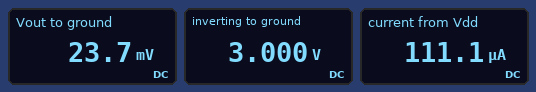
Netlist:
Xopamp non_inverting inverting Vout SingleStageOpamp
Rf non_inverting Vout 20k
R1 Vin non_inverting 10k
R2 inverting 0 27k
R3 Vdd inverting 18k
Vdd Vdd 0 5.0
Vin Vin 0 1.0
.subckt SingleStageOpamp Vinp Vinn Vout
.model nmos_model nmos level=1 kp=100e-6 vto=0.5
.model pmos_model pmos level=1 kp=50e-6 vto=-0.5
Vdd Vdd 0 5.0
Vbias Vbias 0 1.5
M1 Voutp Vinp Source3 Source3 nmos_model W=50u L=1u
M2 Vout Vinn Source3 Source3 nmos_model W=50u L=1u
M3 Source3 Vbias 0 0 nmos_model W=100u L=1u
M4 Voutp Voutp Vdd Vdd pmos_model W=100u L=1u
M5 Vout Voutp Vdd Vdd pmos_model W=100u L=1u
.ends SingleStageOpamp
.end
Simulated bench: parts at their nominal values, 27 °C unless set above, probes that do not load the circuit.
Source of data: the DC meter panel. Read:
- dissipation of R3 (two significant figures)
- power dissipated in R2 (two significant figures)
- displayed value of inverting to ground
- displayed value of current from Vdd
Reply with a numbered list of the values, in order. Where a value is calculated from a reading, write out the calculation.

1. (5 V - 3 V)^2 / 18 kΩ = 220 µW
2. (3 V)^2 / 27 kΩ = 330 µW
3. 3.000 V
4. 111.1 µA
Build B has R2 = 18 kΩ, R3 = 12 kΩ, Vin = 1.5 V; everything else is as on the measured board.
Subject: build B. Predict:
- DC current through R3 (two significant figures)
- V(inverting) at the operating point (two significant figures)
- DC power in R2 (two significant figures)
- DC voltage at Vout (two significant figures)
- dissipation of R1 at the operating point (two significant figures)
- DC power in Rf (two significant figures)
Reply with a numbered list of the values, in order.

1. 170 µA
2. 3.0 V
3. 500 µW
4. 150 mV
5. 20 µW
6. 40 µW
